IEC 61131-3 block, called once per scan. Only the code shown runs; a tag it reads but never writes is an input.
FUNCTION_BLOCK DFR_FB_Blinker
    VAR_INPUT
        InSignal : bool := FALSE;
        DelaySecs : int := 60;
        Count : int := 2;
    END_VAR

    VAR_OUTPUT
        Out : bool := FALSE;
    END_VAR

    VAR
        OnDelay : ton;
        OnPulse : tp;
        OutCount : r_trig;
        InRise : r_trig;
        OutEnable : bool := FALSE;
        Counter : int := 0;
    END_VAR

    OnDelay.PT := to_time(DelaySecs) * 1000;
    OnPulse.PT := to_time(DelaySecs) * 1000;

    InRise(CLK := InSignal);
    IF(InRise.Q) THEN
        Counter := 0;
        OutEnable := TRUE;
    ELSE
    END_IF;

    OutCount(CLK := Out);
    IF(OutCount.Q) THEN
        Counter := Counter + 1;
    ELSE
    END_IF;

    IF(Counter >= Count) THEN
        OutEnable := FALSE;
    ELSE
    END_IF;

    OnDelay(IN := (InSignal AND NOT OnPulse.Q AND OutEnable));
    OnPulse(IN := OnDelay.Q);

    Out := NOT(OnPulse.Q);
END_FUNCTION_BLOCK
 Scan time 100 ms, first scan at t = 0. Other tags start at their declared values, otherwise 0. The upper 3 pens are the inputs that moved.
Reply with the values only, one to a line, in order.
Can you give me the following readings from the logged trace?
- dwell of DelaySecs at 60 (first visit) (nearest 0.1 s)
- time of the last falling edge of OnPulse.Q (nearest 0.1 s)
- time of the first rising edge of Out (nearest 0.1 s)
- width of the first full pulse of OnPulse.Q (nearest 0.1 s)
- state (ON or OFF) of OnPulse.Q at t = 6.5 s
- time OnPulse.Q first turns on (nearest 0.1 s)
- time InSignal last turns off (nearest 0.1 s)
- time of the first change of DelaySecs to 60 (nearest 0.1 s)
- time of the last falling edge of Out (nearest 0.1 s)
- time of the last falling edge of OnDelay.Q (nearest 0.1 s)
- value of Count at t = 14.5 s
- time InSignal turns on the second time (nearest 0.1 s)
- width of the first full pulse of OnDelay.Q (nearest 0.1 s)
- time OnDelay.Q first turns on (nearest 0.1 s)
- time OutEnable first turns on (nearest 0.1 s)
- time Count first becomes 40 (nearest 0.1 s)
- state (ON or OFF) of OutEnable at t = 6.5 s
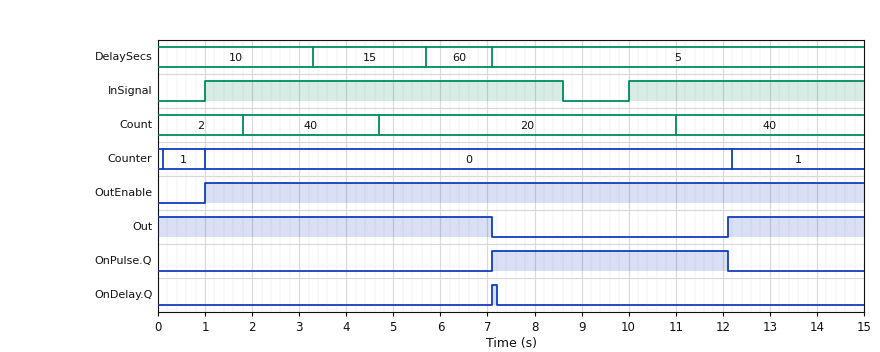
1.4 s
12.1 s
12.1 s
5.0 s
OFF
7.1 s
8.6 s
5.7 s
7.1 s
7.2 s
40
10.0 s
0.1 s
7.1 s
1.0 s
1.8 s
ON
